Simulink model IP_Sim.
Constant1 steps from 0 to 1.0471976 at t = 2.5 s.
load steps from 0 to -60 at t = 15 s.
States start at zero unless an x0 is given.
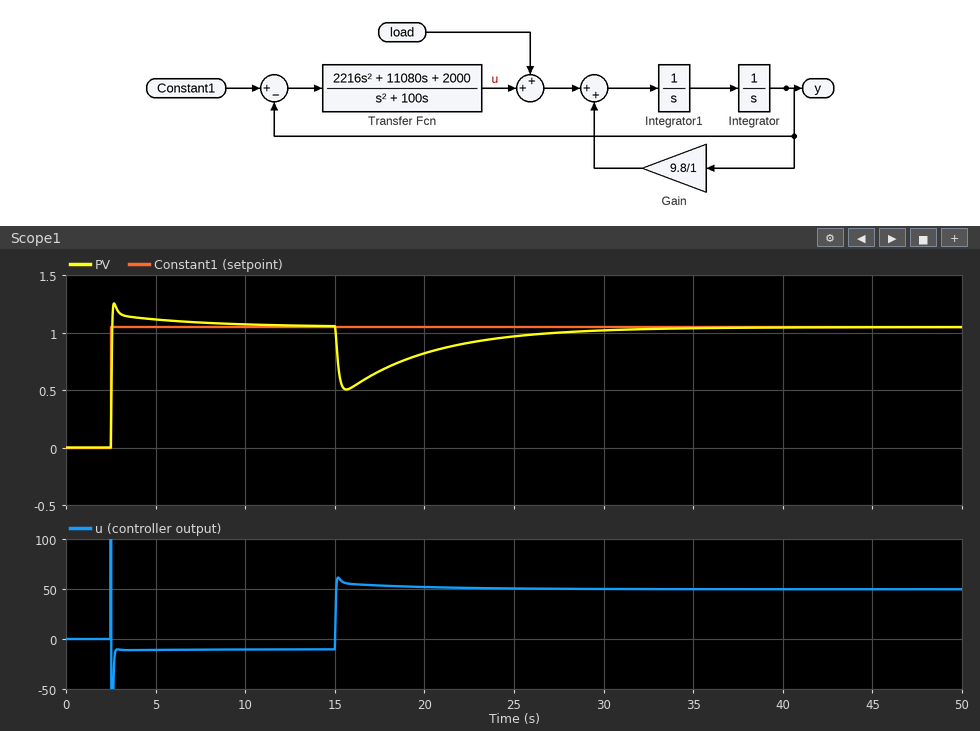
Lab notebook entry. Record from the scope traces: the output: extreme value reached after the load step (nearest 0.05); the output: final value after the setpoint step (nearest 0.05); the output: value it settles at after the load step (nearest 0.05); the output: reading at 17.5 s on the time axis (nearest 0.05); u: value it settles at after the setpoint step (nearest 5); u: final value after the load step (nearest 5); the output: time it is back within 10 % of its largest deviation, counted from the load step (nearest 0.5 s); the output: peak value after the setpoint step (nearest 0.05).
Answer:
0.50
1.05
1.05
0.65
-10
50
12.0 s
1.25
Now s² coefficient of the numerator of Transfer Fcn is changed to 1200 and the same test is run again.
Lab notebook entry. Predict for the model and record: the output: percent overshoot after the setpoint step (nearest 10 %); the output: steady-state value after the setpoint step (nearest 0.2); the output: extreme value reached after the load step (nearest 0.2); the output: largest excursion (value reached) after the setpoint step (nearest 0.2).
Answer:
40 %
1.0
0.4
1.4
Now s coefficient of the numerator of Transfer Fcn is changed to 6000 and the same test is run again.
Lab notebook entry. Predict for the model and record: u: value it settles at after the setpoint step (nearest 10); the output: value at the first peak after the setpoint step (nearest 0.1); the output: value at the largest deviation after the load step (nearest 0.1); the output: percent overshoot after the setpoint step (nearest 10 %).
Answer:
-10
1.2
0.1
20 %
